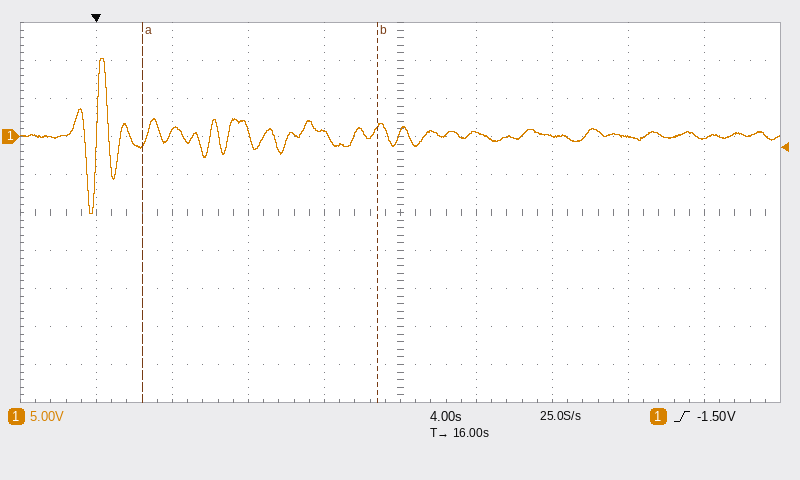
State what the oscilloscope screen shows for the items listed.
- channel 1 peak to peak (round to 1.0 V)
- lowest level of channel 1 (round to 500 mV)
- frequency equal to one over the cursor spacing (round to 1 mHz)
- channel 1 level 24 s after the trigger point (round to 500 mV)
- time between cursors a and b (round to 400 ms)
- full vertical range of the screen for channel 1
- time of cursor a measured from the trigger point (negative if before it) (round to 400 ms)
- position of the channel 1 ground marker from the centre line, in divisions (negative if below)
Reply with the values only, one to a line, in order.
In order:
20.0 V
-10.0 V
81 mHz
0.0 V
12.4 s
50 V
+2.4 s
+2.0 div
